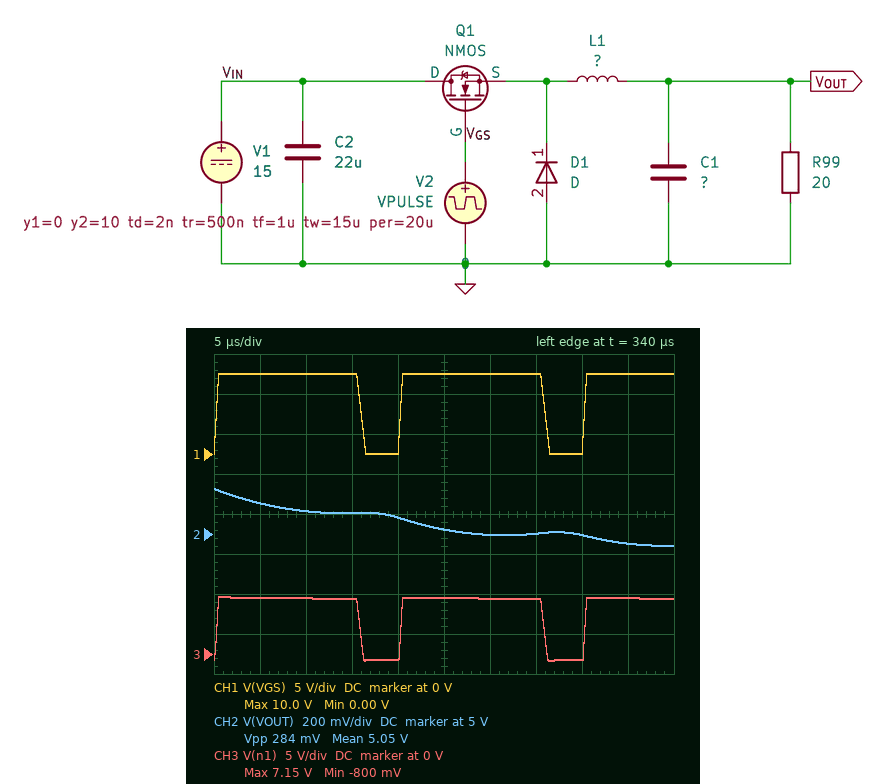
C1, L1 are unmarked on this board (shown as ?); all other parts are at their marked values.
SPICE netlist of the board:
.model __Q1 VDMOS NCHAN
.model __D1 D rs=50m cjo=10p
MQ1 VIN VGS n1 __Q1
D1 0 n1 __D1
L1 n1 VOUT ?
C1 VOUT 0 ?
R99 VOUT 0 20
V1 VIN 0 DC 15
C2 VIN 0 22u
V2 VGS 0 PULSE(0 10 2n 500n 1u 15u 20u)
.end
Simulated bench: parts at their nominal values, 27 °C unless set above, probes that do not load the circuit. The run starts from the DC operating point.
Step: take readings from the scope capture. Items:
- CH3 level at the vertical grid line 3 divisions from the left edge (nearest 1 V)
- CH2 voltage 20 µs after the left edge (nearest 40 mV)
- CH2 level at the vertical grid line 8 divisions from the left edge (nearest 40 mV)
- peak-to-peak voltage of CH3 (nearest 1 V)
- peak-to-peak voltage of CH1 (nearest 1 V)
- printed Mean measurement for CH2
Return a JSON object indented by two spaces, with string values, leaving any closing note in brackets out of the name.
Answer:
{
  "CH3 level at the vertical grid line 3 divisions from the left edge": "7 V",
  "CH2 voltage 20 µs after the left edge": "5.08 V",
  "CH2 level at the vertical grid line 8 divisions from the left edge": "5.00 V",
  "peak-to-peak voltage of CH3": "8 V",
  "peak-to-peak voltage of CH1": "10 V",
  "printed Mean measurement for CH2": "5.05 V"
}
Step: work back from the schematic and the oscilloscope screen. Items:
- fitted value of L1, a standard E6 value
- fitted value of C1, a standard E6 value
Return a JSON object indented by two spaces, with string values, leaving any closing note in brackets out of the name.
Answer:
{
  "fitted value of L1, a standard E6 value": "100 µH",
  "fitted value of C1, a standard E6 value": "15 µF"
}
